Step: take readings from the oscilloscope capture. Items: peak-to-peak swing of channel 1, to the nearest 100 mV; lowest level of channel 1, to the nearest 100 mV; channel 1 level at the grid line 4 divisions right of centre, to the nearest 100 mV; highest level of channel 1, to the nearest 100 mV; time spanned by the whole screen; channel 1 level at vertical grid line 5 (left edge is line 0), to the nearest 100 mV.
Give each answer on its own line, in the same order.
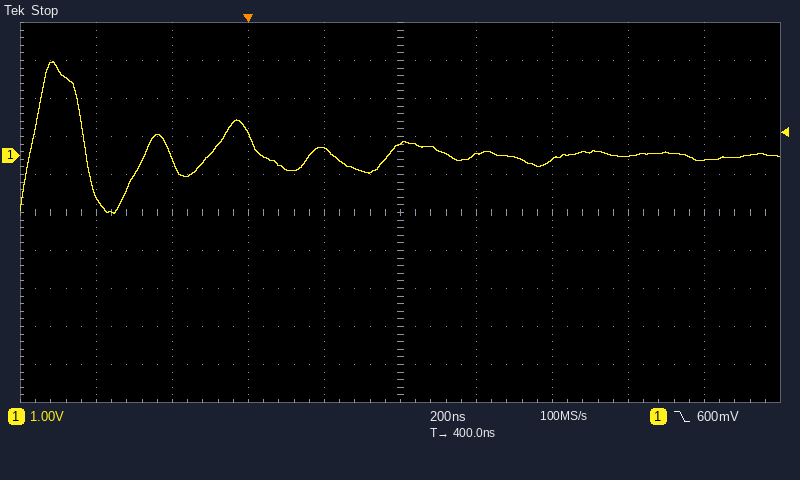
4.0 V
-1.5 V
-100 mV
2.5 V
2 µs
300 mV
